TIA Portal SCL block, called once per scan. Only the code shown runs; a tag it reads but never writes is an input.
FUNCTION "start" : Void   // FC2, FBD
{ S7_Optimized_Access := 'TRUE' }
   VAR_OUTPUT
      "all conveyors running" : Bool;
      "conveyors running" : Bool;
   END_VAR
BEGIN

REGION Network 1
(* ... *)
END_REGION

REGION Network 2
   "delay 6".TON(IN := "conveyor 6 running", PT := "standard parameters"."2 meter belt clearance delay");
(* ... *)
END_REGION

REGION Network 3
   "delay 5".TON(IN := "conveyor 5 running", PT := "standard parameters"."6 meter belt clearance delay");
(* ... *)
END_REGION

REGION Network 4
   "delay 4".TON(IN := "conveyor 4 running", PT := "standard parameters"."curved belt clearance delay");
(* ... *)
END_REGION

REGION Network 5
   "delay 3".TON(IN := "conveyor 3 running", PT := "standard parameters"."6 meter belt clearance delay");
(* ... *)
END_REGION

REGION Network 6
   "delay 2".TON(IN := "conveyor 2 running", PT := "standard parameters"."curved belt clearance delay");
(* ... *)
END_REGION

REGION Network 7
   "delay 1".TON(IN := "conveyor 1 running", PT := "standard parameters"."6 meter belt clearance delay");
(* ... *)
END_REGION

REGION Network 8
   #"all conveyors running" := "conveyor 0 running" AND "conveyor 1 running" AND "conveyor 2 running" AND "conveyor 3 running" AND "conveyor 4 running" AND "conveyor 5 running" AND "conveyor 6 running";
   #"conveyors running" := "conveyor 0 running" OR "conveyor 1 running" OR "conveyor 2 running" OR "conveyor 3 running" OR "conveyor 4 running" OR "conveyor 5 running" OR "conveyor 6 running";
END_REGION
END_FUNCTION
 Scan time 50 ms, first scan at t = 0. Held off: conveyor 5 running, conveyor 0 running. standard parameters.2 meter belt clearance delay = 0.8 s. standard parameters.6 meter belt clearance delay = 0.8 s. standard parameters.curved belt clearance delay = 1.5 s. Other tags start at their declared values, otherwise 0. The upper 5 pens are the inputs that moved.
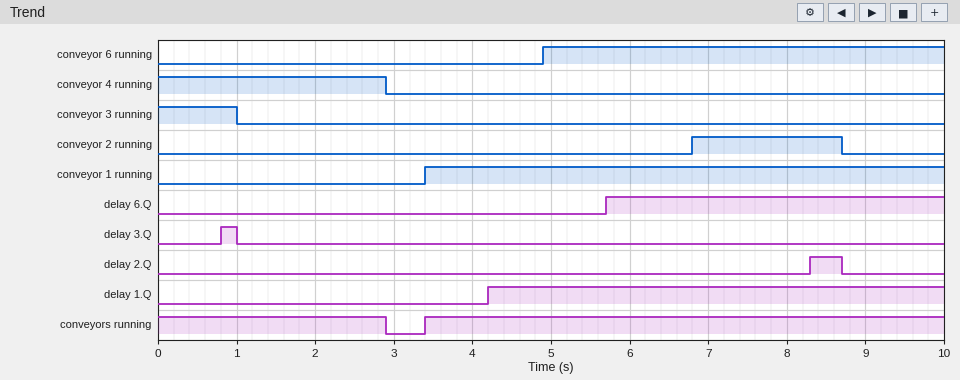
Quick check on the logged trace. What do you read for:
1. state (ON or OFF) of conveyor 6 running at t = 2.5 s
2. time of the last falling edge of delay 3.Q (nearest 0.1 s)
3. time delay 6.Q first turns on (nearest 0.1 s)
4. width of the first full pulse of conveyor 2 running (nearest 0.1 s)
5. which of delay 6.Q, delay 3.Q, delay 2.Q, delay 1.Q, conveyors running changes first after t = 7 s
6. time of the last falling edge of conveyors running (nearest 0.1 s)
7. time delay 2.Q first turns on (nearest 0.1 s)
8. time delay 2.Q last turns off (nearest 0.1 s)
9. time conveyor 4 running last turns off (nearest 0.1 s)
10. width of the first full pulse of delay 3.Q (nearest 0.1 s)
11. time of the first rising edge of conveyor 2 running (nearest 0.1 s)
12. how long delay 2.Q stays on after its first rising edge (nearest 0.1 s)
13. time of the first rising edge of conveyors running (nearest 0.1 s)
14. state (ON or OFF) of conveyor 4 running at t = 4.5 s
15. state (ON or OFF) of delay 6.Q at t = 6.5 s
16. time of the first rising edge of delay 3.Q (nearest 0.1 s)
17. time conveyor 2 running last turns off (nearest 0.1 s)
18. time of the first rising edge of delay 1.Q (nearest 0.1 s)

OFF
1.0 s
5.7 s
1.9 s
delay 2.Q
2.9 s
8.3 s
8.7 s
2.9 s
0.2 s
6.8 s
0.4 s
3.4 s
OFF
ON
0.8 s
8.7 s
4.2 s
